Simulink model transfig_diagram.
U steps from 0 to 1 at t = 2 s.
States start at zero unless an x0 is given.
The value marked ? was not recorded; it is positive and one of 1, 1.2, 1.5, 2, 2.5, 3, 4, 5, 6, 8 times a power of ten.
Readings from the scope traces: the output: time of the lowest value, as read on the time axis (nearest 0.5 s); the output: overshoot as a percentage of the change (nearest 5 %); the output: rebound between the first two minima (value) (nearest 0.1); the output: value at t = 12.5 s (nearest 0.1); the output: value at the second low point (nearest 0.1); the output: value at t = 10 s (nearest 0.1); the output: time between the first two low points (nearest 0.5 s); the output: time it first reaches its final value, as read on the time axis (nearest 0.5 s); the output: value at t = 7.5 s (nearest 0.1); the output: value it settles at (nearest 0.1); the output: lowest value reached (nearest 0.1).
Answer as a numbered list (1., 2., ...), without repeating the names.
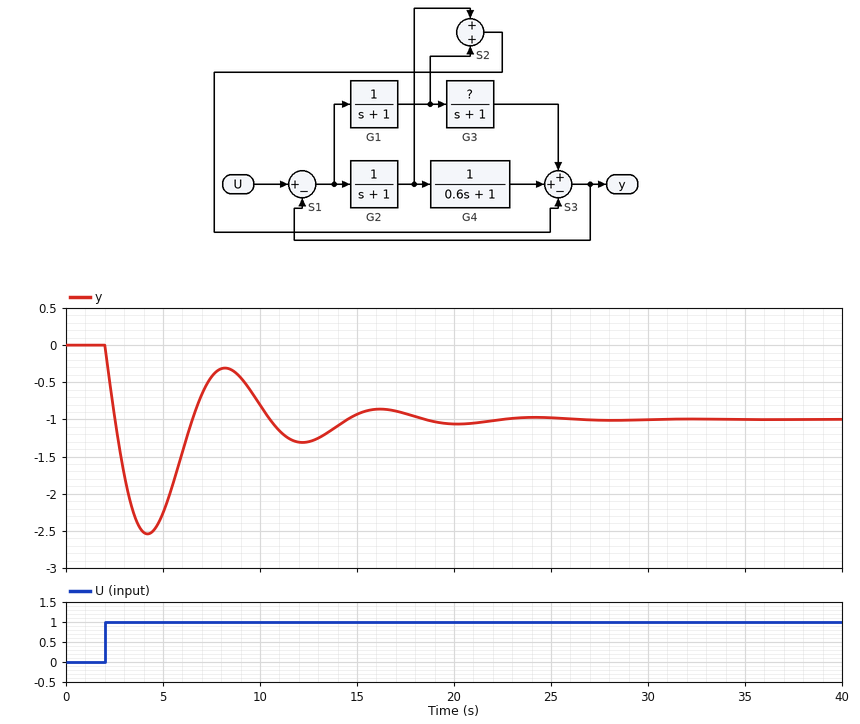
1. 4.0 s
2. 155 %
3. -0.3
4. -1.3
5. -1.3
6. -0.8
7. 8.0 s
8. 2.5 s
9. -0.4
10. -1.0
11. -2.5
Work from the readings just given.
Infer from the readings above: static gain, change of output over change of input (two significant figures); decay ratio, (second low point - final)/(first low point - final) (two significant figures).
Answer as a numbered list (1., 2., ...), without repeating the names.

1. -1.0
2. 0.20
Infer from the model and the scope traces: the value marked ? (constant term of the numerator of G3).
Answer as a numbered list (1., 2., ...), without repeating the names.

1. 0.5
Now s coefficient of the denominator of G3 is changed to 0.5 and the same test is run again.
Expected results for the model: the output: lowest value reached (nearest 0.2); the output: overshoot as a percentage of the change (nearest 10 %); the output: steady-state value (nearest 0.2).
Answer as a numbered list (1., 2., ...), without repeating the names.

1. -2.0
2. 90 %
3. -1.0
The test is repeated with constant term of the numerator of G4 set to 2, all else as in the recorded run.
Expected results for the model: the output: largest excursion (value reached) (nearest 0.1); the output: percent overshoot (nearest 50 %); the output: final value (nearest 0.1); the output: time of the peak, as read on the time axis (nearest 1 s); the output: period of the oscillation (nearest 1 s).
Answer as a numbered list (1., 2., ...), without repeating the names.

1. 1.0
2. 200 %
3. 0.3
4. 5 s
5. 4 s
